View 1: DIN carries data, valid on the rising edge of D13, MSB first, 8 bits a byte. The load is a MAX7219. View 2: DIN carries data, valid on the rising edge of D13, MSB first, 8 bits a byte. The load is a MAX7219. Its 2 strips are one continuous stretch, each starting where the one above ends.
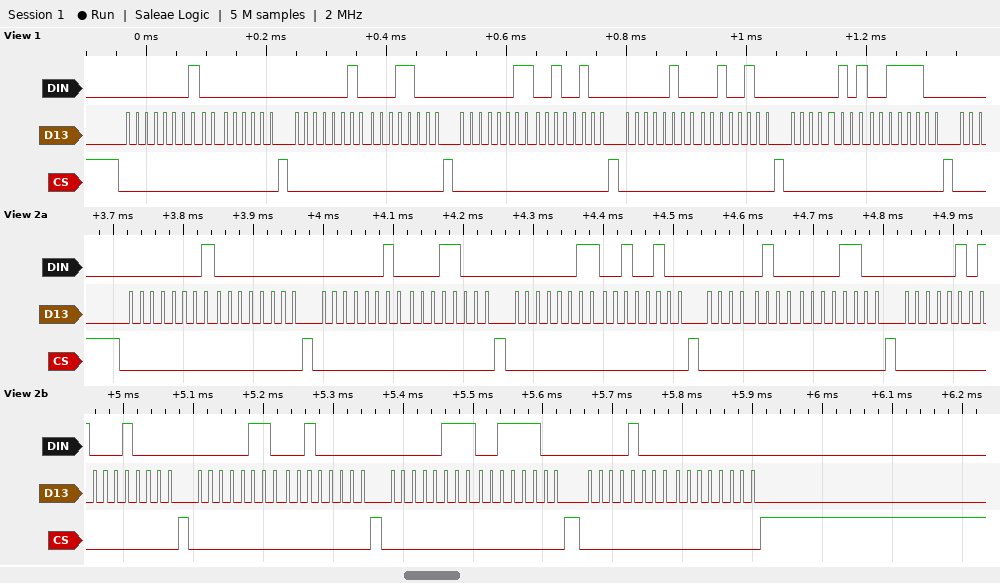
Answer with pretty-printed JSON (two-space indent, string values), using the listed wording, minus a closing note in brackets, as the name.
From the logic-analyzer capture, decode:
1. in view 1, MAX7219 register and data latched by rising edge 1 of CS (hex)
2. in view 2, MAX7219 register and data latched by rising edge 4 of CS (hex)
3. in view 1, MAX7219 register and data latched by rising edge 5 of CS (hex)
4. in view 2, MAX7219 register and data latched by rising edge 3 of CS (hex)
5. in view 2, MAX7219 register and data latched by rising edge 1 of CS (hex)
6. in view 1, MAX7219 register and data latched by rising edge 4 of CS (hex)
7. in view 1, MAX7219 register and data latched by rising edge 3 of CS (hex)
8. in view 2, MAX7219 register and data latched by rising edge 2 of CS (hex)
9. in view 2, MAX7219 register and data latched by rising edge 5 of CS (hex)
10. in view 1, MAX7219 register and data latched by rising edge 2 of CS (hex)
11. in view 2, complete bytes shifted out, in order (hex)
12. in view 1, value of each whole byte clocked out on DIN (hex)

{
  "in view 1, MAX7219 register and data latched by rising edge 1 of CS": "register 0x1, data 0x00",
  "in view 2, MAX7219 register and data latched by rising edge 4 of CS": "register 0x4, data 0x0C",
  "in view 1, MAX7219 register and data latched by rising edge 5 of CS": "register 0x5, data 0x3C",
  "in view 2, MAX7219 register and data latched by rising edge 3 of CS": "register 0x3, data 0x24",
  "in view 2, MAX7219 register and data latched by rising edge 1 of CS": "register 0x1, data 0x00",
  "in view 1, MAX7219 register and data latched by rising edge 4 of CS": "register 0x4, data 0x24",
  "in view 1, MAX7219 register and data latched by rising edge 3 of CS": "register 0x3, data 0x24",
  "in view 2, MAX7219 register and data latched by rising edge 2 of CS": "register 0x2, data 0x18",
  "in view 2, MAX7219 register and data latched by rising edge 5 of CS": "register 0x5, data 0x10",
  "in view 1, MAX7219 register and data latched by rising edge 2 of CS": "register 0x2, data 0x18",
  "in view 2, complete bytes shifted out, in order": "01 00 02 18 03 24 04 0C 05 10 06 20 07 3C 08 00",
  "in view 1, value of each whole byte clocked out on DIN": "0x01 0x00 0x02 0x18 0x03 0x24 0x04 0x24 0x05 0x3C"
}
